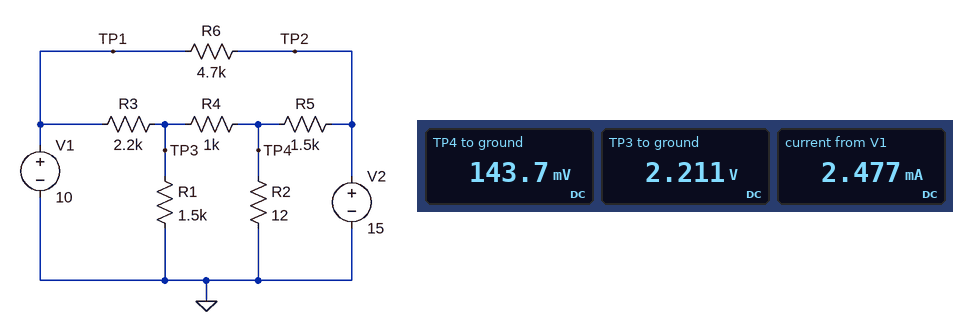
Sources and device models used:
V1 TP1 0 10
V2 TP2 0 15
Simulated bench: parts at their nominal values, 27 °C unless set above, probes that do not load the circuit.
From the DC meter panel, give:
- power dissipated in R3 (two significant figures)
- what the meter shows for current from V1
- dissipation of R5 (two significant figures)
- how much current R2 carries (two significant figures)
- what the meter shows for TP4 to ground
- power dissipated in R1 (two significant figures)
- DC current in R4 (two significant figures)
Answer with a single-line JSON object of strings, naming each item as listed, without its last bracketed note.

{"power dissipated in R3": "28 mW", "what the meter shows for current from V1": "2.477 mA", "dissipation of R5": "150 mW", "how much current R2 carries": "12 mA", "what the meter shows for TP4 to ground": "143.7 mV", "power dissipated in R1": "3.3 mW", "DC current in R4": "2.1 mA"}
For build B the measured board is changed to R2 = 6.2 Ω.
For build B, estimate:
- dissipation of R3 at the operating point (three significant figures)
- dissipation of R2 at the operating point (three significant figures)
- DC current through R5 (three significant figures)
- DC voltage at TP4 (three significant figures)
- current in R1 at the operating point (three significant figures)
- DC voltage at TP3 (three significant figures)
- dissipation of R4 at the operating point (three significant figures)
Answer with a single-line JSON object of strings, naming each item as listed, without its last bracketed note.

{"dissipation of R3 at the operating point": "27.8 mW", "dissipation of R2 at the operating point": "901 µW", "DC current through R5": "9.95 mA", "DC voltage at TP4": "74.7 mV", "current in R1 at the operating point": "1.45 mA", "DC voltage at TP3": "2.18 V", "dissipation of R4 at the operating point": "4.42 mW"}
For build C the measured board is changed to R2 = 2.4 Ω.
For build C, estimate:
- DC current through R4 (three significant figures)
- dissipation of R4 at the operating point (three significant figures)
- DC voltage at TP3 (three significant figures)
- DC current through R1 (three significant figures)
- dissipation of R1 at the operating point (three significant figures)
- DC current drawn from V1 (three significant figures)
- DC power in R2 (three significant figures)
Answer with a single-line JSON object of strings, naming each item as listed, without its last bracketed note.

{"DC current through R4": "2.13 mA", "dissipation of R4 at the operating point": "4.53 mW", "DC voltage at TP3": "2.16 V", "DC current through R1": "1.44 mA", "dissipation of R1 at the operating point": "3.10 mW", "DC current drawn from V1": "2.50 mA", "DC power in R2": "352 µW"}
